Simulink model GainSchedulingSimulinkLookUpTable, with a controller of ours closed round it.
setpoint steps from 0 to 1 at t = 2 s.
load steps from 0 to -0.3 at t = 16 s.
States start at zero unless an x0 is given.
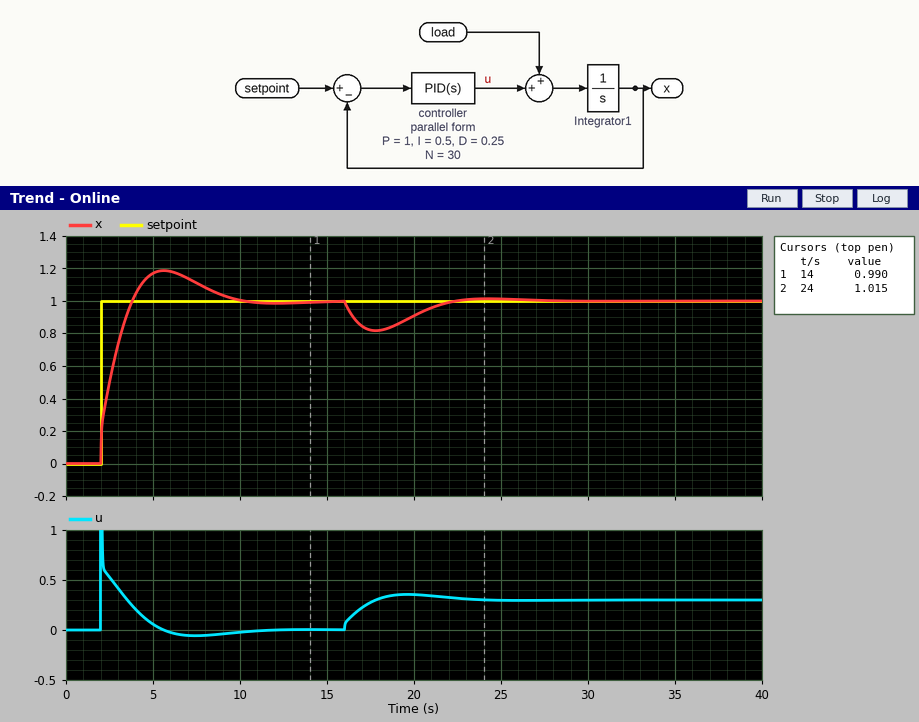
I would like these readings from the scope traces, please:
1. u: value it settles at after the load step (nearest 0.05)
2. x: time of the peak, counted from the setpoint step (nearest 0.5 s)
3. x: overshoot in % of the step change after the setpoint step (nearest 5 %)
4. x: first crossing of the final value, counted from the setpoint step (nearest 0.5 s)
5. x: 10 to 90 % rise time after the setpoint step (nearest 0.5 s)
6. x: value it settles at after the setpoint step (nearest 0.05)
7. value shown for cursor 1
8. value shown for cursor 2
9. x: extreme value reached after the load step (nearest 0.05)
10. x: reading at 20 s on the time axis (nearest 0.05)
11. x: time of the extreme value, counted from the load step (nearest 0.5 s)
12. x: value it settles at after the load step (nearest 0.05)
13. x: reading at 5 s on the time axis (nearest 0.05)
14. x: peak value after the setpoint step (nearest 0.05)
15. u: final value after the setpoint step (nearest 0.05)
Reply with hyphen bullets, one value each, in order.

- 0.30
- 3.5 s
- 20 %
- 2.0 s
- 1.5 s
- 1.00
- 0.990
- 1.015
- 0.80
- 0.90
- 2.0 s
- 1.00
- 1.15
- 1.20
- 0.00
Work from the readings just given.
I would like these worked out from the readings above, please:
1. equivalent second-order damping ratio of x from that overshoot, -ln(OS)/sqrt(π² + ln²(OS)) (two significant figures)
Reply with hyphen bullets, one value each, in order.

- 0.46
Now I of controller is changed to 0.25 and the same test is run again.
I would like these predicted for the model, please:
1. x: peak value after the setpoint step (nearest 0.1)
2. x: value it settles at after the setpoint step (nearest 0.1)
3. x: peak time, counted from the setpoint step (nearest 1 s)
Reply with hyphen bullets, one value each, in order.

- 1.1
- 1.0
- 5 s
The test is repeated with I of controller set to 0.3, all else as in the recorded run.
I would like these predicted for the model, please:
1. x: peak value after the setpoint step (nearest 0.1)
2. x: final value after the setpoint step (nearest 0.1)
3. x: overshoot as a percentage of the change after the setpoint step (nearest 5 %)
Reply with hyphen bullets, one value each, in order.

- 1.1
- 1.0
- 15 %
